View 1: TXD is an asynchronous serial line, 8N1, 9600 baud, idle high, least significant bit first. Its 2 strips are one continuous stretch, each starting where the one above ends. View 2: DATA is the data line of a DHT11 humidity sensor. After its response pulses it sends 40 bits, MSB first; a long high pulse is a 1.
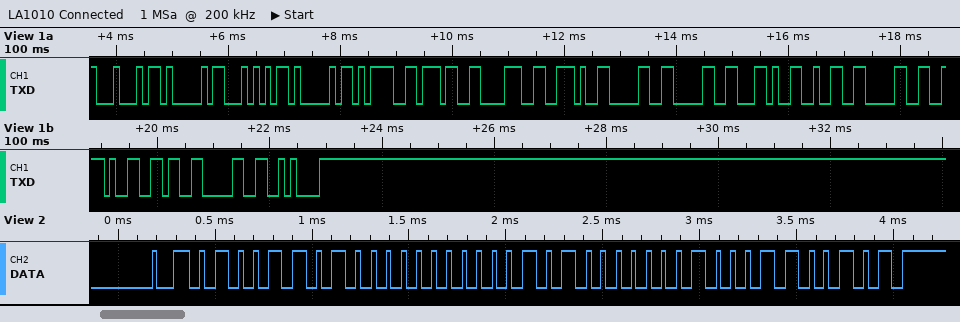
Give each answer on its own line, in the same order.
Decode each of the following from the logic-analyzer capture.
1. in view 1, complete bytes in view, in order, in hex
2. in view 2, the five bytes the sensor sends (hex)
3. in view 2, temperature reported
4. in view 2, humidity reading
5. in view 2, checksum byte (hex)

44 41 54 41 3D 37 38 2E 30 30 2C 32 30 2E 36 30 0A
4D 00 14 04 65
20.4 °C
77 %
0x65
